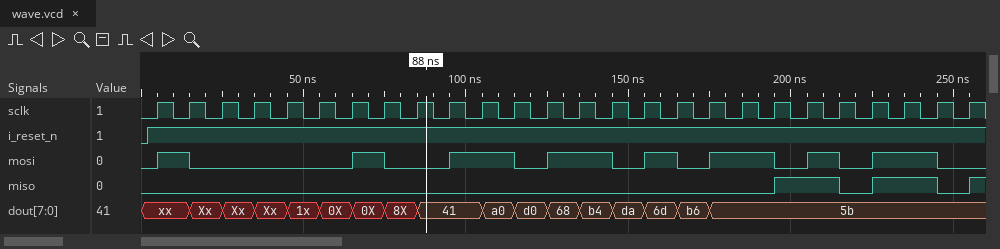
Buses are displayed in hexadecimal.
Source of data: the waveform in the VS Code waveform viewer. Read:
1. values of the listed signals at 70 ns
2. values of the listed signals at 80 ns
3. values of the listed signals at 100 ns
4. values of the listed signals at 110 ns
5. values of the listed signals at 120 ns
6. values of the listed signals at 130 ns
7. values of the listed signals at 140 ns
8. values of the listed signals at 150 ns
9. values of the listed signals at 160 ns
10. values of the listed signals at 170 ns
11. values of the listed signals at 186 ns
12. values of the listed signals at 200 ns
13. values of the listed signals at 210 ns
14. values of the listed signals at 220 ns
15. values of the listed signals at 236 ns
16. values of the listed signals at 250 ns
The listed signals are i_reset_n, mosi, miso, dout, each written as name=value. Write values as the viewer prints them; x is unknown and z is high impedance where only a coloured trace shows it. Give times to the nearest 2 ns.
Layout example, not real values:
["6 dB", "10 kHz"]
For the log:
["i_reset_n=1, mosi=1, miso=0, dout=0X", "i_reset_n=1, mosi=0, miso=0, dout=8X", "i_reset_n=1, mosi=1, miso=0, dout=41", "i_reset_n=1, mosi=1, miso=0, dout=a0", "i_reset_n=1, mosi=0, miso=0, dout=d0", "i_reset_n=1, mosi=1, miso=0, dout=68", "i_reset_n=1, mosi=1, miso=0, dout=b4", "i_reset_n=1, mosi=0, miso=0, dout=da", "i_reset_n=1, mosi=1, miso=0, dout=6d", "i_reset_n=1, mosi=0, miso=0, dout=b6", "i_reset_n=1, mosi=1, miso=0, dout=5b", "i_reset_n=1, mosi=0, miso=1, dout=5b", "i_reset_n=1, mosi=1, miso=1, dout=5b", "i_reset_n=1, mosi=0, miso=0, dout=5b", "i_reset_n=1, mosi=1, miso=1, dout=5b", "i_reset_n=1, mosi=0, miso=0, dout=5b"]
